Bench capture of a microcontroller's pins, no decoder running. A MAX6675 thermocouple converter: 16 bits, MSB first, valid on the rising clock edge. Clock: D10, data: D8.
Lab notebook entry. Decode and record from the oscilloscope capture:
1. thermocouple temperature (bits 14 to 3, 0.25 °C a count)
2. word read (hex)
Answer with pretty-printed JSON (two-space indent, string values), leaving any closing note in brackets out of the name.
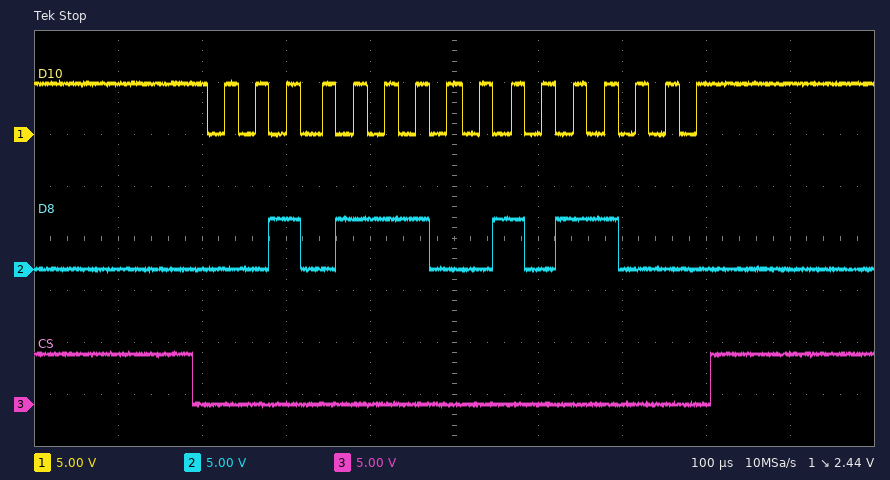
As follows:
{
  "thermocouple temperature": "370.75 °C",
  "word read": "0x2E58"
}
